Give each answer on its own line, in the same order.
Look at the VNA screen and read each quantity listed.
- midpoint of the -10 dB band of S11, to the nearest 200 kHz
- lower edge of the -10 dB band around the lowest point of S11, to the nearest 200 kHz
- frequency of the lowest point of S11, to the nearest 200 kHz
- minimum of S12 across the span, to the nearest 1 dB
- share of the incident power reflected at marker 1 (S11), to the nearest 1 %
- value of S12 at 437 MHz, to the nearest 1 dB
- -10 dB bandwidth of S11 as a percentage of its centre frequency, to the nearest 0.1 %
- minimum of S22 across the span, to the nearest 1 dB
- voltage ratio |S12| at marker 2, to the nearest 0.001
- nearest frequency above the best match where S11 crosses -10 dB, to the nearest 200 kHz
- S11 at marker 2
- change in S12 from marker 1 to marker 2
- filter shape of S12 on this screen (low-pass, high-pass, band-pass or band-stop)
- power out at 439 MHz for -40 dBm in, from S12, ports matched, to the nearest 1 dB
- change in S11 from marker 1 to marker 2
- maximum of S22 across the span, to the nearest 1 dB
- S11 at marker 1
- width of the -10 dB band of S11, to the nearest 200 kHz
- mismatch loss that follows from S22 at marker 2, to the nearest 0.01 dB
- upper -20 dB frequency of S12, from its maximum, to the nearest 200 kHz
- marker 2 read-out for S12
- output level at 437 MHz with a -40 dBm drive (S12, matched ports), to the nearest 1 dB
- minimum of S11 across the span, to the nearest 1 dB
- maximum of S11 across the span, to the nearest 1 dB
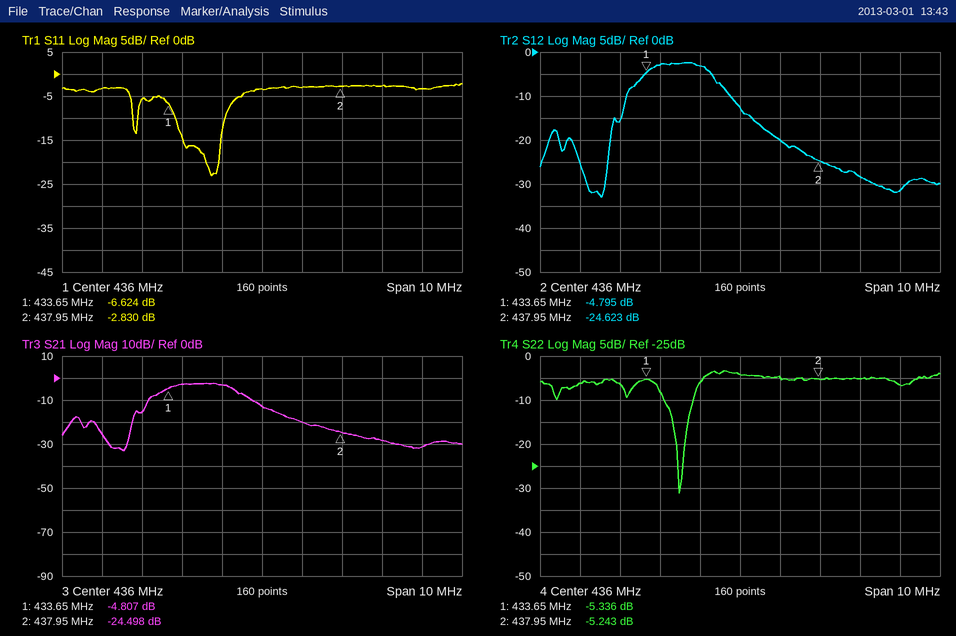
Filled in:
434.4 MHz
433.8 MHz
434.8 MHz
-33 dB
22 %
-20 dB
0.3 %
-31 dB
0.059
435.0 MHz
-2.830 dB
-19.828 dB
band-pass
-68 dBm
3.794 dB
-3 dB
-6.624 dB
1.2 MHz
1.54 dB
437.6 MHz
-24.623 dB
-60 dBm
-23 dB
-2 dB
